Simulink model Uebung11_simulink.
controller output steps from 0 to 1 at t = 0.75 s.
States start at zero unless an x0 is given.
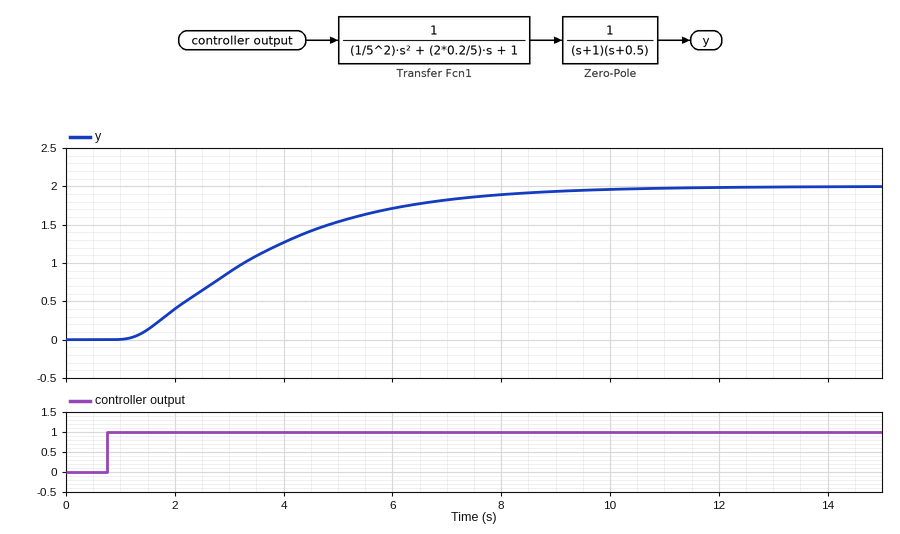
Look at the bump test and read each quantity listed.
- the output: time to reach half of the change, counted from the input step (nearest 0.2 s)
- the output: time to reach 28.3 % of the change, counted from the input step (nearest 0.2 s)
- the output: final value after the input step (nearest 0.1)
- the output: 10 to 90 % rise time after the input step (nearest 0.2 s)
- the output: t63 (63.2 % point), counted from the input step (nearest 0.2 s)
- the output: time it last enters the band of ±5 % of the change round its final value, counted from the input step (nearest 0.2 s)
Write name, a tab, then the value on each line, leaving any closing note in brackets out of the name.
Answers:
the output: time to reach half of the change, counted from the input step	2.6 s
the output: time to reach 28.3 % of the change, counted from the input step	1.6 s
the output: final value after the input step	2.0
the output: 10 to 90 % rise time after the input step	5.2 s
the output: t63 (63.2 % point), counted from the input step	3.2 s
the output: time it last enters the band of ±5 % of the change round its final value, counted from the input step	7.4 s
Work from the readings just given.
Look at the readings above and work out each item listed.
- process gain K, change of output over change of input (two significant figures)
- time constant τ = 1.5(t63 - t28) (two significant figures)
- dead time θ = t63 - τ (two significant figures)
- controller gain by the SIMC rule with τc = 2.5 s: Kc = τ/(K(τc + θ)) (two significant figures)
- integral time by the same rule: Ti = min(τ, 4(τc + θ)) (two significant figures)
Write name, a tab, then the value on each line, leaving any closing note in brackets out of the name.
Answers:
process gain K, change of output over change of input	2.0
time constant τ = 1.5(t63 - t28)	2.4 s
dead time θ = t63 - τ	0.80 s
controller gain by the SIMC rule with τc = 2.5 s: Kc = τ/(K(τc + θ))	0.36
integral time by the same rule: Ti = min(τ, 4(τc + θ))	2.4 s
